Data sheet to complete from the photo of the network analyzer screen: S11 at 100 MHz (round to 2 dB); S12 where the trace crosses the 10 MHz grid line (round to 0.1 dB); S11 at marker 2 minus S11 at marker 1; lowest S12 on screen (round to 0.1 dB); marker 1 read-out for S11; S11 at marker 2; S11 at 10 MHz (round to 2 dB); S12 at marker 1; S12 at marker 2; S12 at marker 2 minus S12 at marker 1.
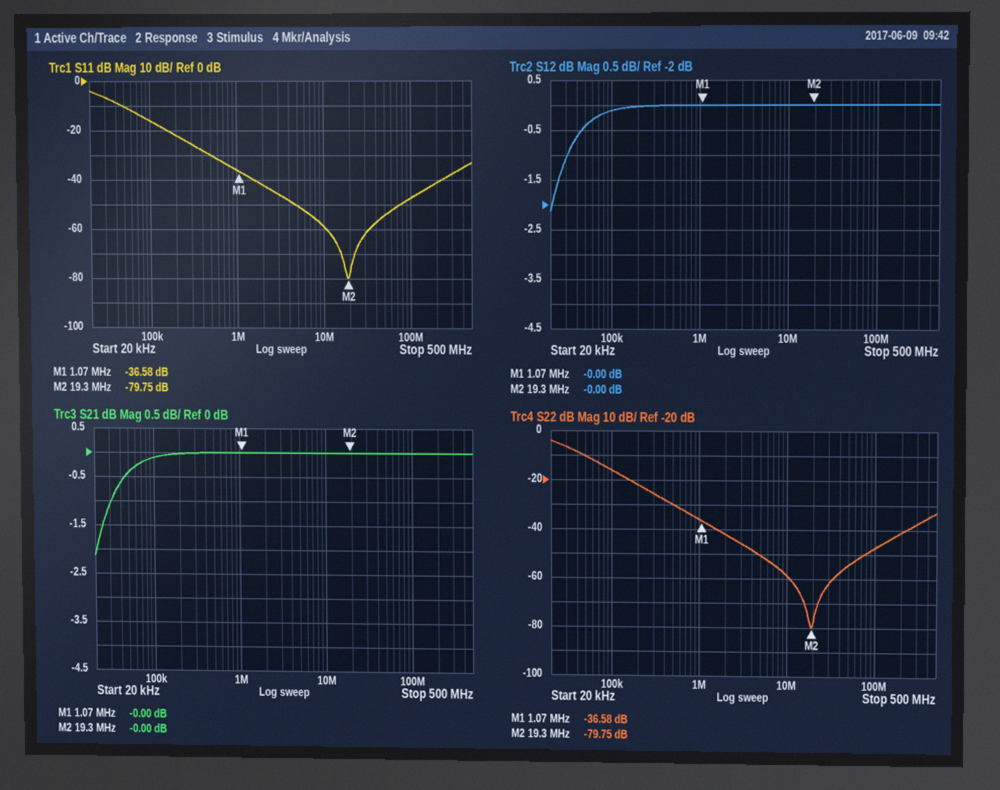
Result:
-48 dB
0.0 dB
-43.17 dB
-2.1 dB
-36.58 dB
-79.75 dB
-58 dB
-0.00 dB
-0.00 dB
0.00 dB
